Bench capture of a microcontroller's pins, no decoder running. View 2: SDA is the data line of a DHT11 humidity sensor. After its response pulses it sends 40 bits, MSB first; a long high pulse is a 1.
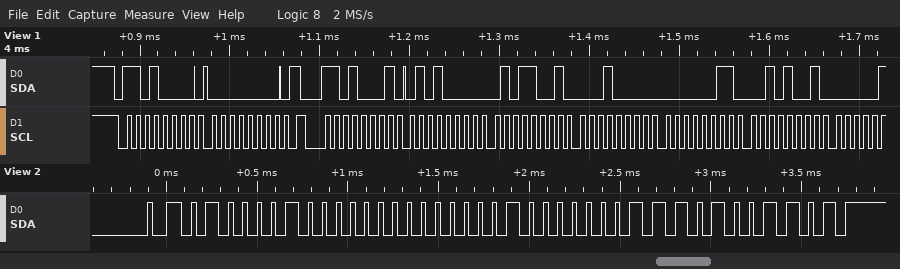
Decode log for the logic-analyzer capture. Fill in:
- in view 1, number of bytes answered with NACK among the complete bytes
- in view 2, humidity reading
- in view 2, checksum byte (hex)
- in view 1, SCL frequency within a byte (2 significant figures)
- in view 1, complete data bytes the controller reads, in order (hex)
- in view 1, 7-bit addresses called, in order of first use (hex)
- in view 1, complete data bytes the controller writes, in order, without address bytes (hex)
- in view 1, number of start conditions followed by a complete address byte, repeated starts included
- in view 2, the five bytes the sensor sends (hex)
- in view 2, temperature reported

0
66 %
0x4D
100 kHz
50 59 10 03 29
0x68
00
2
42 00 04 07 4D
4.7 °C
